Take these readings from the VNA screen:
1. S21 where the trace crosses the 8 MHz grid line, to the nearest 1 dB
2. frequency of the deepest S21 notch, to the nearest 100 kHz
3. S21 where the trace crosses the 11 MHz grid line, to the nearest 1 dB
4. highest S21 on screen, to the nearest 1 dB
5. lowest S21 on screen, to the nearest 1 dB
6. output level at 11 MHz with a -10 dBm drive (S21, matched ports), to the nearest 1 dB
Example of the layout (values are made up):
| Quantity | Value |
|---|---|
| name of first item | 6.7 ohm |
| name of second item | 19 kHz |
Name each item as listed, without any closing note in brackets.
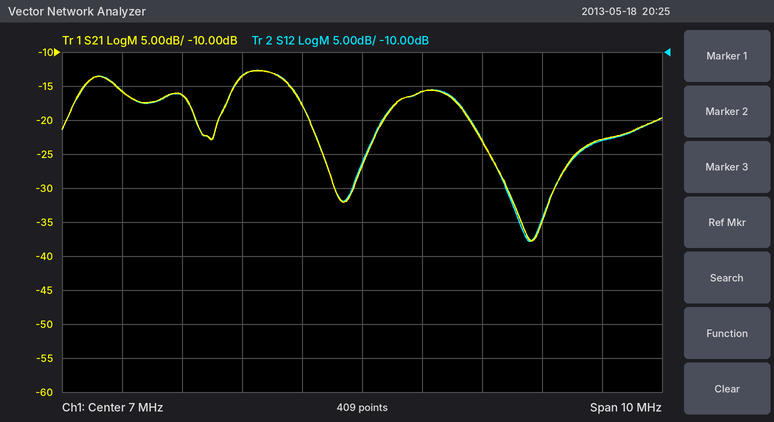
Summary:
| Quantity | Value |
|---|---|
| S21 where the trace crosses the 8 MHz grid line, to the nearest 1 dB | -16 dB |
| frequency of the deepest S21 notch, to the nearest 100 kHz | 9.8 MHz |
| S21 where the trace crosses the 11 MHz grid line, to the nearest 1 dB | -23 dB |
| highest S21 on screen, to the nearest 1 dB | -13 dB |
| lowest S21 on screen, to the nearest 1 dB | -38 dB |
| output level at 11 MHz with a -10 dBm drive (S21, matched ports), to the nearest 1 dB | -33 dBm |
